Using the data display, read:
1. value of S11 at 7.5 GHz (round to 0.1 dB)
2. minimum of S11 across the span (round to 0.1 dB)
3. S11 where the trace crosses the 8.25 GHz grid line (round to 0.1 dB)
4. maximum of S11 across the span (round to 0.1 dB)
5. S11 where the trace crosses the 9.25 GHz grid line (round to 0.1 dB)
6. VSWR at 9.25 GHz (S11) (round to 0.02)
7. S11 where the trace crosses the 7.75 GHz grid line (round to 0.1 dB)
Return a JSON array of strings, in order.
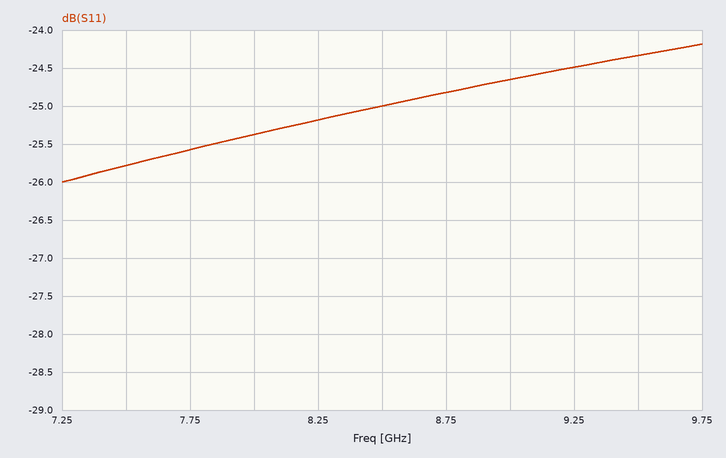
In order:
["-25.8 dB", "-26.0 dB", "-25.2 dB", "-24.2 dB", "-24.5 dB", "1.12", "-25.6 dB"]
